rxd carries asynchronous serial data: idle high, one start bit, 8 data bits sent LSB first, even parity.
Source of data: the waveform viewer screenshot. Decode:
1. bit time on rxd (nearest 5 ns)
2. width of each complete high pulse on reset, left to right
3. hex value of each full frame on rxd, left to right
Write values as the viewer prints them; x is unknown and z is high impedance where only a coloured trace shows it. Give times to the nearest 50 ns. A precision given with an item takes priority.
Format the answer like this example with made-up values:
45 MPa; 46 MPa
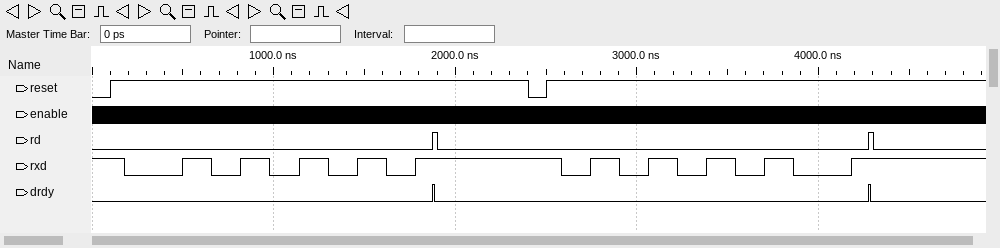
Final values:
160 ns; 2300 ns; AA, 55
